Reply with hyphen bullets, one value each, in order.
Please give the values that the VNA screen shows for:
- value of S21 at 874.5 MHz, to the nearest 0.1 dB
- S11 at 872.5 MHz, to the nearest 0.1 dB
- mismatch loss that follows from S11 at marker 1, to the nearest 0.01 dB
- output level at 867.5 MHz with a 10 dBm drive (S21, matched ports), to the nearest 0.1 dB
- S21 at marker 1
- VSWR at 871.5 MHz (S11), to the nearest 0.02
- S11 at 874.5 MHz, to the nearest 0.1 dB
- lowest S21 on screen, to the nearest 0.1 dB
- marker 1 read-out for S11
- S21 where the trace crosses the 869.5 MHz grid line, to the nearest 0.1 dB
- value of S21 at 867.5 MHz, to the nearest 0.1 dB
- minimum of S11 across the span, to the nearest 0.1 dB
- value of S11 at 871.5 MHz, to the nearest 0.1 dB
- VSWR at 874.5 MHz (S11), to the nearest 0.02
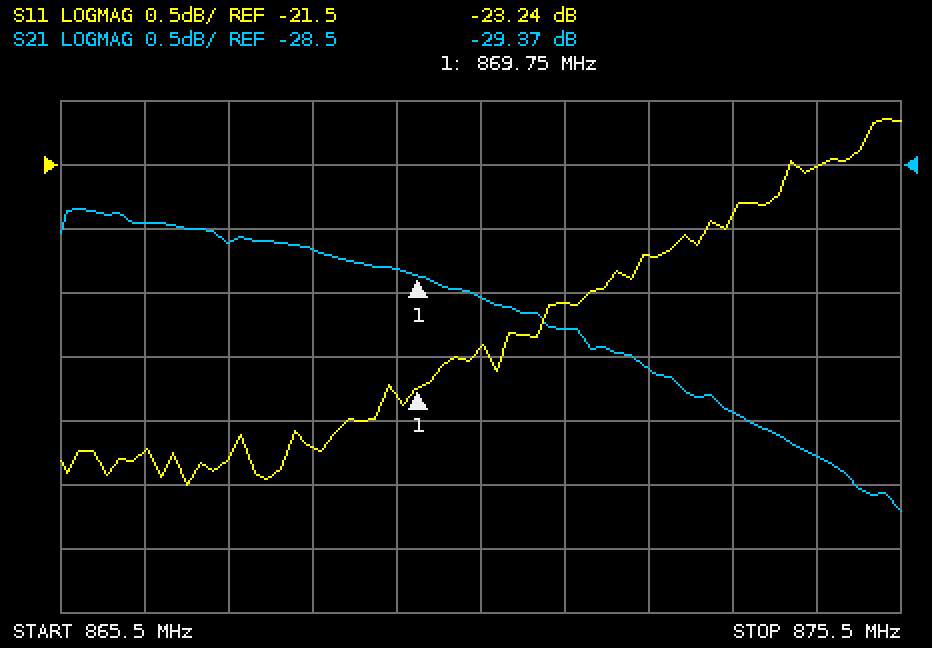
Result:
- -30.8 dB
- -22.2 dB
- 0.02 dB
- -19.1 dBm
- -29.37 dB
- 1.16
- -21.5 dB
- -31.2 dB
- -23.24 dB
- -29.3 dB
- -29.1 dB
- -24.0 dB
- -22.6 dB
- 1.18
